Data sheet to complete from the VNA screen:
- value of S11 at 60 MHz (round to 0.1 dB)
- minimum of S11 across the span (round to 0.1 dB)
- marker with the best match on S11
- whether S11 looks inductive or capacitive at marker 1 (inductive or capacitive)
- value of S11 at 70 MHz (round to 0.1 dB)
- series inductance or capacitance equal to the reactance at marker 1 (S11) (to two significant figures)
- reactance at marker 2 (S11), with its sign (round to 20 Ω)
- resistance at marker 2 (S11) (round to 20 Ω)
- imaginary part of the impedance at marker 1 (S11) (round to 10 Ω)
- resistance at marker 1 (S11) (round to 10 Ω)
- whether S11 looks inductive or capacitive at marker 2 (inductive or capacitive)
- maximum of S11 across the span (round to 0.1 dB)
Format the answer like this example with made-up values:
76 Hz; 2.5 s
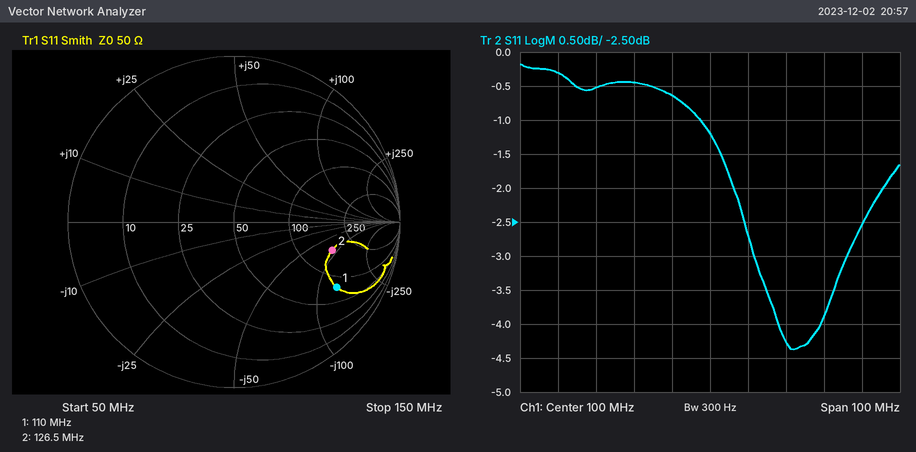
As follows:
-0.3 dB; -4.4 dB; marker 2; capacitive; -0.5 dB; 11 pF; -80 Ω; 160 Ω; -130 Ω; 80 Ω; capacitive; -0.2 dB
